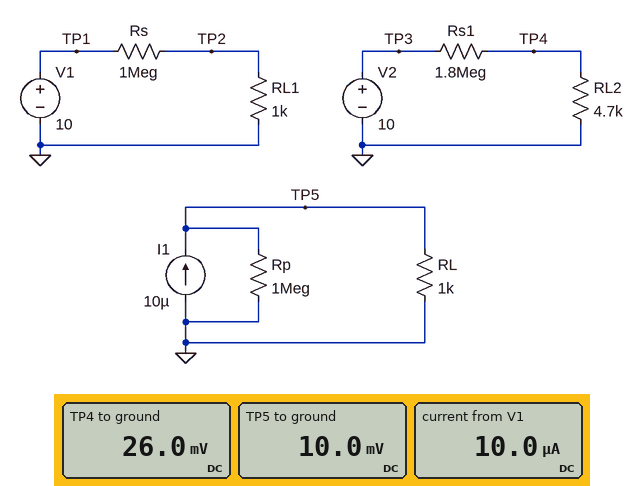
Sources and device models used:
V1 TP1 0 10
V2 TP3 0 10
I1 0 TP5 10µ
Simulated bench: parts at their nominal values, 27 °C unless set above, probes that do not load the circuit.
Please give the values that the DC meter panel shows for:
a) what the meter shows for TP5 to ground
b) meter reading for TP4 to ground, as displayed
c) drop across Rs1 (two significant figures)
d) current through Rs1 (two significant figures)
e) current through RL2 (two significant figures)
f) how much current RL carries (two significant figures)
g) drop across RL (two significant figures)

10.0 mV
26.0 mV
10 V
5.5 µA
5.5 µA
10 µA
10 mV
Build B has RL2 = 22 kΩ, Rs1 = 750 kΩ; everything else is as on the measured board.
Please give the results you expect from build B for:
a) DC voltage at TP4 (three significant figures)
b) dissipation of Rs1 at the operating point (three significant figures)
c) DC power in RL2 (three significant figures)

285 mV
126 µW
3.69 µW
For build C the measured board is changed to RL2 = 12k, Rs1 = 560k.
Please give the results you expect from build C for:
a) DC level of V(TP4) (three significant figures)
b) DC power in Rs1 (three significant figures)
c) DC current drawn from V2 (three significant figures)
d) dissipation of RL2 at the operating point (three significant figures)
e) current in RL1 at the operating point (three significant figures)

210 mV
171 µW
17.5 µA
3.67 µW
9.99 µA
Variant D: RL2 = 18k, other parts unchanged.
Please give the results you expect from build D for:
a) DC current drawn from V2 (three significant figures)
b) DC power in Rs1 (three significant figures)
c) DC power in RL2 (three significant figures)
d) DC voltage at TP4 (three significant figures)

5.50 µA
54.5 µW
545 nW
99.0 mV
